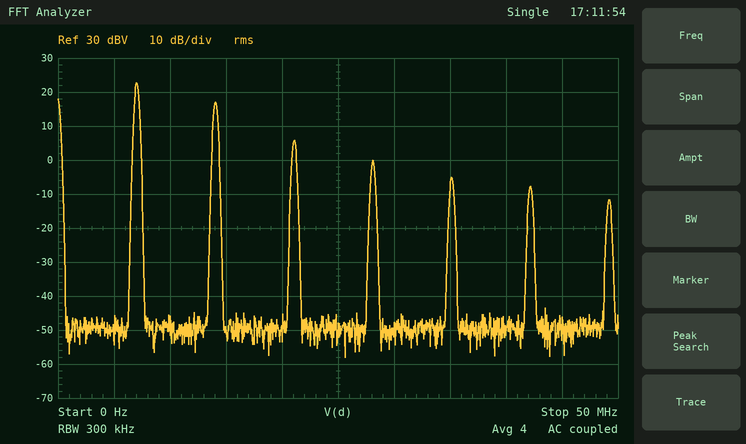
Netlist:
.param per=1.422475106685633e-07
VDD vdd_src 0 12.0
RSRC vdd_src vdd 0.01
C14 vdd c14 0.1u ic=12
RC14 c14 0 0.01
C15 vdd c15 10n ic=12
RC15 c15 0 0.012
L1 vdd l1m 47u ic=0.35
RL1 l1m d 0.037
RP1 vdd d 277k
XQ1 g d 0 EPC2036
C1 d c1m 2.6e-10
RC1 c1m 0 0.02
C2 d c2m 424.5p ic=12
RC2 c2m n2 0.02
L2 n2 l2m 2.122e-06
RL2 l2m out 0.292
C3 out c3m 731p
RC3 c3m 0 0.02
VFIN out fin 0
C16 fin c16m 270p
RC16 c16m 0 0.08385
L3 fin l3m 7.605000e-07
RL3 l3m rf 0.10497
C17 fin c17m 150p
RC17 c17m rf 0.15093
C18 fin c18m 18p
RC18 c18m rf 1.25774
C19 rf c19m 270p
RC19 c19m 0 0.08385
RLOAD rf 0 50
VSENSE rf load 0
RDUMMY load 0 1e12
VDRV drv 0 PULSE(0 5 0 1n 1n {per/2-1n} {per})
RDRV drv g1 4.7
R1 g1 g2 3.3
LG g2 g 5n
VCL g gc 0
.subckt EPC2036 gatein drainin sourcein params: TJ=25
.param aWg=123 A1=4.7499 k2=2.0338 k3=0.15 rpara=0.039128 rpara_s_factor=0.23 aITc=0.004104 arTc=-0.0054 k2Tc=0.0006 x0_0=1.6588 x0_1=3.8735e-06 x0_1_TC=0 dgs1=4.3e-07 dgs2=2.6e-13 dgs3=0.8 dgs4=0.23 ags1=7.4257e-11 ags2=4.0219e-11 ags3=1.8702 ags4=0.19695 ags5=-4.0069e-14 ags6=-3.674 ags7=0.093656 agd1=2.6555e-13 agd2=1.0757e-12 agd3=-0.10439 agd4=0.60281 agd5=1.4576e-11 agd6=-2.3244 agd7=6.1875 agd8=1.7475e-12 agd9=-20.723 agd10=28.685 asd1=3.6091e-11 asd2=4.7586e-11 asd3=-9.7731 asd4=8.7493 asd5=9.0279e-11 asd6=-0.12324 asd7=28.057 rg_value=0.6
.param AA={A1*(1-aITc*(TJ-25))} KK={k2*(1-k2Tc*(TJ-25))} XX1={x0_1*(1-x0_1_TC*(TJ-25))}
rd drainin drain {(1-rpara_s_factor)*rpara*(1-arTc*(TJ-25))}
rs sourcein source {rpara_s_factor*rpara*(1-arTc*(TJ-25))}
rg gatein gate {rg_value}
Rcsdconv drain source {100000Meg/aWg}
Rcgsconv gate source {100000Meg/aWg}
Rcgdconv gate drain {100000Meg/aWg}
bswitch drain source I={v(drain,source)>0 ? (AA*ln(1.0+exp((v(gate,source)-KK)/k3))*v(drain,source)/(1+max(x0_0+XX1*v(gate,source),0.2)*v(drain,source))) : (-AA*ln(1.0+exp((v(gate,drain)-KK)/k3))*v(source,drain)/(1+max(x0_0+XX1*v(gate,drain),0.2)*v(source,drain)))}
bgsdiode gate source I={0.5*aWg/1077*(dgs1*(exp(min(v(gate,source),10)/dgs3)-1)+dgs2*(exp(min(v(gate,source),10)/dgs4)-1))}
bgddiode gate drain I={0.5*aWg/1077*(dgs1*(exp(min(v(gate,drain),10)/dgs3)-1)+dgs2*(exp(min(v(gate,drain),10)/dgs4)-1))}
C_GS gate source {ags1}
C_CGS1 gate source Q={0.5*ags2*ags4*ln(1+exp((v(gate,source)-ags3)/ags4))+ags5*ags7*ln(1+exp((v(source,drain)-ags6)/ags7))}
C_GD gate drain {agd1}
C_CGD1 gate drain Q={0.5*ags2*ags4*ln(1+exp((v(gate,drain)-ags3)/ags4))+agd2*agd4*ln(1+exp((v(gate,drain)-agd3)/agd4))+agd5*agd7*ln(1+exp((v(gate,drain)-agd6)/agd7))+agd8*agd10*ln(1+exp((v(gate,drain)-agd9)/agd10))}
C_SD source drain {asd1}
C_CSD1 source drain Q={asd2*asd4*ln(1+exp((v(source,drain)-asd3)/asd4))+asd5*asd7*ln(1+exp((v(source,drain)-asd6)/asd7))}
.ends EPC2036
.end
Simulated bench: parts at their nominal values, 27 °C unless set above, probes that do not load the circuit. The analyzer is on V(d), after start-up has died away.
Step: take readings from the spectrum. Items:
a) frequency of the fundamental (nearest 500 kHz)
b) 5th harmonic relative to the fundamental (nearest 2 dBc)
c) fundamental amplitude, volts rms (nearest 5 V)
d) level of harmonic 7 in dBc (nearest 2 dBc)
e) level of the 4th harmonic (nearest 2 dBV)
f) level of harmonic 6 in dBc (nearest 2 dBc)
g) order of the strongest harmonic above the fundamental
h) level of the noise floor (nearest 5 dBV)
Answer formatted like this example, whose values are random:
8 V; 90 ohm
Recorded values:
7.0 MHz; -28 dBc; 15 V; -34 dBc; 0 dBV; -30 dBc; 2; -50 dBV
